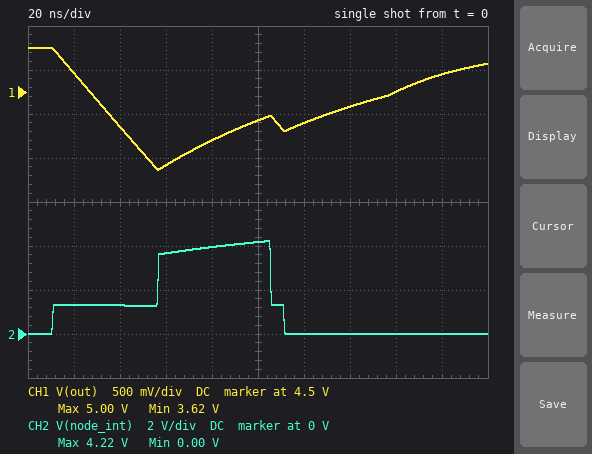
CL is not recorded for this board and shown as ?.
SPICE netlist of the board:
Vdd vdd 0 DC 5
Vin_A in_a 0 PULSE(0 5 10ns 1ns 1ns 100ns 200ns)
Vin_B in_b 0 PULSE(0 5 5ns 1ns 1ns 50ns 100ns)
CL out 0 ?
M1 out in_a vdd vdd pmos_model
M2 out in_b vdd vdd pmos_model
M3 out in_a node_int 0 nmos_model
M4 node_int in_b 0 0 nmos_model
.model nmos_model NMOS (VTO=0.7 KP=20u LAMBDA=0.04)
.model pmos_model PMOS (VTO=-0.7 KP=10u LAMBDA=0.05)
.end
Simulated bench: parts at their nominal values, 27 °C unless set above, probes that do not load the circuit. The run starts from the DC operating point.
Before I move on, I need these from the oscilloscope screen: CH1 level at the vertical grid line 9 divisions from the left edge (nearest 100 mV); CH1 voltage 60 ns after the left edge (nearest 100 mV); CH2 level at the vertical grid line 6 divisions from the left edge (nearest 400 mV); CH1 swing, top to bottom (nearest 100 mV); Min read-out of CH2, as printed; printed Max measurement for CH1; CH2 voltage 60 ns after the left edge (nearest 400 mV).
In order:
4.7 V
3.7 V
0 V
1.4 V
0.00 V
5.00 V
3.6 V
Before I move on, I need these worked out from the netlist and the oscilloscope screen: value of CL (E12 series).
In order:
3.3 pF
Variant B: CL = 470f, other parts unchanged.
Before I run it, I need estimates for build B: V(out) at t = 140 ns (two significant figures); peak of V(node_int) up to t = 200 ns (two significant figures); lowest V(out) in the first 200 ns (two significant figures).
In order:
4.9 V
4.3 V
160 mV
